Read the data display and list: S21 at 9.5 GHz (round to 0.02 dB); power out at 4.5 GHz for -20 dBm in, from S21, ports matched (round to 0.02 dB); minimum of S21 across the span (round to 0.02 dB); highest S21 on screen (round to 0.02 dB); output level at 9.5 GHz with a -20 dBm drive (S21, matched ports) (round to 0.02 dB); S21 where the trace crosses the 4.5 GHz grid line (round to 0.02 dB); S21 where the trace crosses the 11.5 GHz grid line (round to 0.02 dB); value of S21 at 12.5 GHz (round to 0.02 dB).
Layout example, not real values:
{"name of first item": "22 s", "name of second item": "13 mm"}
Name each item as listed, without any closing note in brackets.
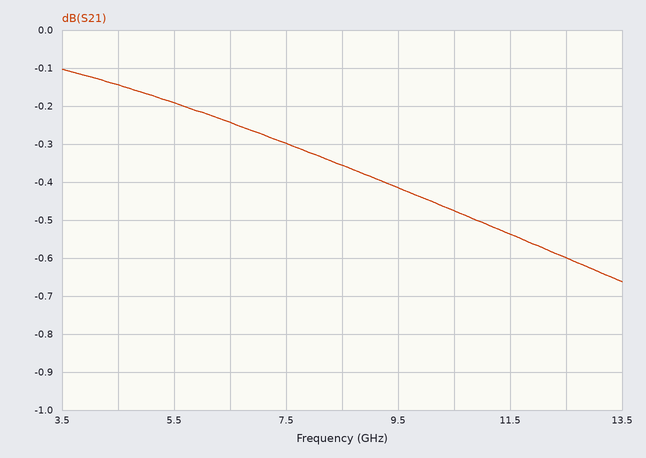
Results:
{"S21 at 9.5 GHz": "-0.42 dB", "power out at 4.5 GHz for -20 dBm in, from S21, ports matched": "-20.14 dBm", "minimum of S21 across the span": "-0.66 dB", "highest S21 on screen": "-0.10 dB", "output level at 9.5 GHz with a -20 dBm drive (S21, matched ports)": "-20.42 dBm", "S21 where the trace crosses the 4.5 GHz grid line": "-0.14 dB", "S21 where the trace crosses the 11.5 GHz grid line": "-0.54 dB", "value of S21 at 12.5 GHz": "-0.60 dB"}
